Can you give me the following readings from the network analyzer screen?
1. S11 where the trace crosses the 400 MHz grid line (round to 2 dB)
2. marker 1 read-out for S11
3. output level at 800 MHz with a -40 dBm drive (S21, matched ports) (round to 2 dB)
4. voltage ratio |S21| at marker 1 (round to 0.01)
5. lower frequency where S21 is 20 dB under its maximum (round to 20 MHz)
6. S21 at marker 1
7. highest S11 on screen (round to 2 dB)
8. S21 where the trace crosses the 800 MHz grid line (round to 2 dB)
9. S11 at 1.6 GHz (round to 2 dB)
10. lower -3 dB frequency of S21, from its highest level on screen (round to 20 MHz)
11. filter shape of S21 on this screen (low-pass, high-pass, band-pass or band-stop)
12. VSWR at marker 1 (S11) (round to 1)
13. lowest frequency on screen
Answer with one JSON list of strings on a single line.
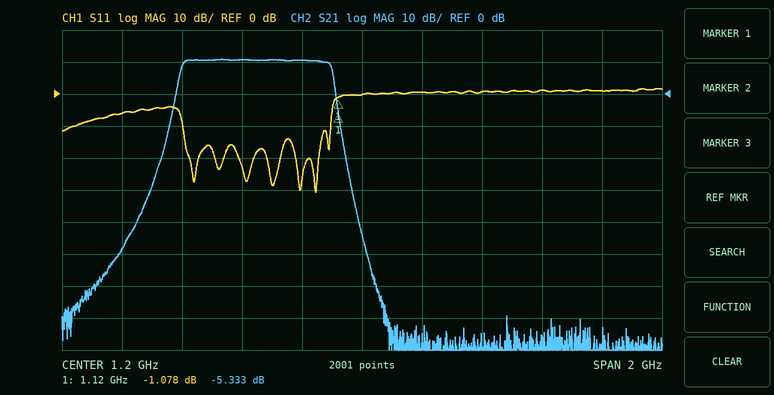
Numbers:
["-6 dB", "-1.078 dB", "-30 dBm", "0.54", "560 MHz", "-5.333 dB", "2 dB", "10 dB", "0 dB", "600 MHz", "band-pass", "16", "200 MHz"]
